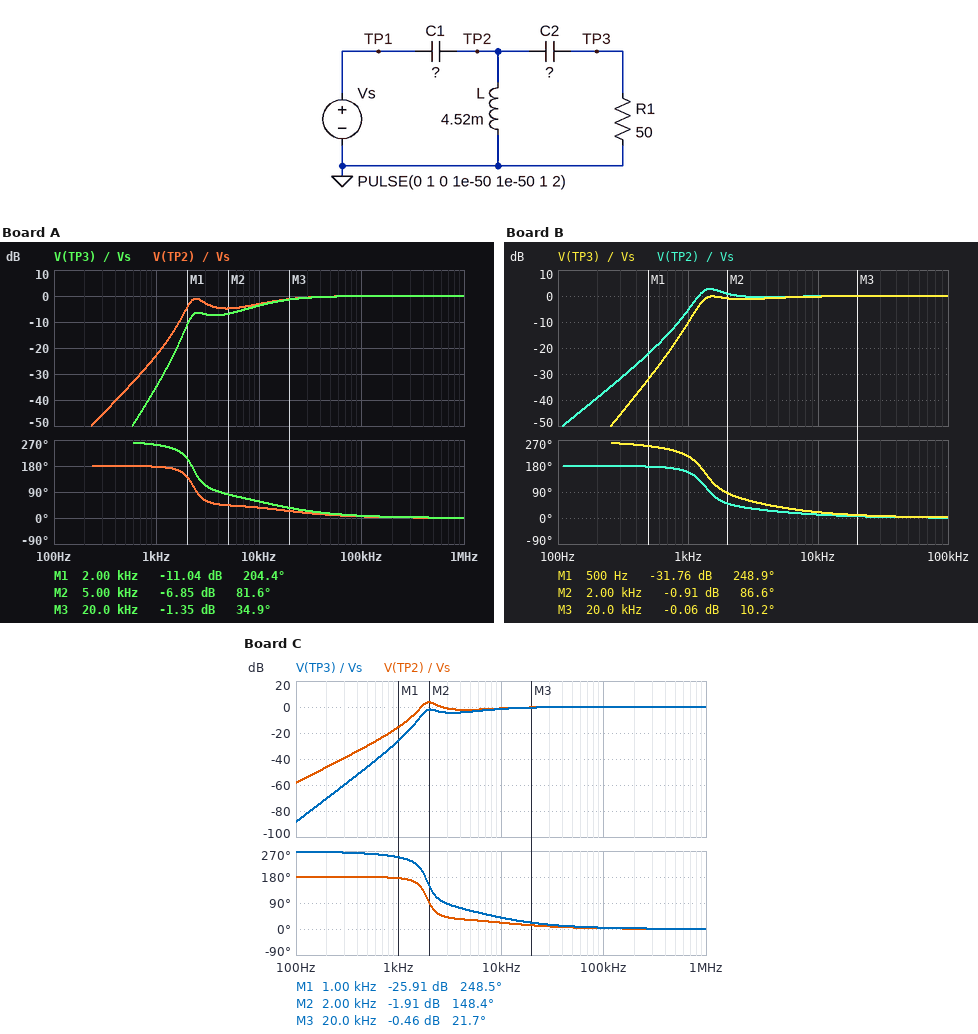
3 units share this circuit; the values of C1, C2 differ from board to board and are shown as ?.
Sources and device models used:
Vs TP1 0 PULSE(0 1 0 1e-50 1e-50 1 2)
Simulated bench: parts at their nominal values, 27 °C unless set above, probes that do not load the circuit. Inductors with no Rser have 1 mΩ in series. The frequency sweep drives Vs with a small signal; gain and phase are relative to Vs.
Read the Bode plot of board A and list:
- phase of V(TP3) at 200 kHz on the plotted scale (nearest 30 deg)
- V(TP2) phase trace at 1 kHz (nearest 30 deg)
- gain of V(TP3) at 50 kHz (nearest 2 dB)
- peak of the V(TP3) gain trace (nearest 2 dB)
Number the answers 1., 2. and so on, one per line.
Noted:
1. 0 deg
2. 180 deg
3. 0 dB
4. 0 dB
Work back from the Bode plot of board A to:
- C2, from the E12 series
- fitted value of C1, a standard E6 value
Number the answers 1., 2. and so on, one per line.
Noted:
1. 820 nF
2. 330 nF
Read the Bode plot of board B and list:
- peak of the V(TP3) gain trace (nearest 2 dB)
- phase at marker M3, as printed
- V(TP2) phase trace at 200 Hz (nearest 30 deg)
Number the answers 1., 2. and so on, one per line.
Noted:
1. 0 dB
2. 10.2 deg
3. 180 deg
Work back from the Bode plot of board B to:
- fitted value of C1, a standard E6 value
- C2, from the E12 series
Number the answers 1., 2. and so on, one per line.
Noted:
1. 1.5 µF
2. 2.2 µF
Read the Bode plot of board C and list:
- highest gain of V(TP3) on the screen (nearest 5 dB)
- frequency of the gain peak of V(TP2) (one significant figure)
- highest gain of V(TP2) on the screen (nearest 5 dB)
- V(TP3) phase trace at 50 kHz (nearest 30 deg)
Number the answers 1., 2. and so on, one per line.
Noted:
1. 0 dB
2. 2 kHz
3. 5 dB
4. 0 deg
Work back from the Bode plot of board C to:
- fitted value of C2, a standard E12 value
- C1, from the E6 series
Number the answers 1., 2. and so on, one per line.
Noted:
1. 1 µF
2. 680 nF
